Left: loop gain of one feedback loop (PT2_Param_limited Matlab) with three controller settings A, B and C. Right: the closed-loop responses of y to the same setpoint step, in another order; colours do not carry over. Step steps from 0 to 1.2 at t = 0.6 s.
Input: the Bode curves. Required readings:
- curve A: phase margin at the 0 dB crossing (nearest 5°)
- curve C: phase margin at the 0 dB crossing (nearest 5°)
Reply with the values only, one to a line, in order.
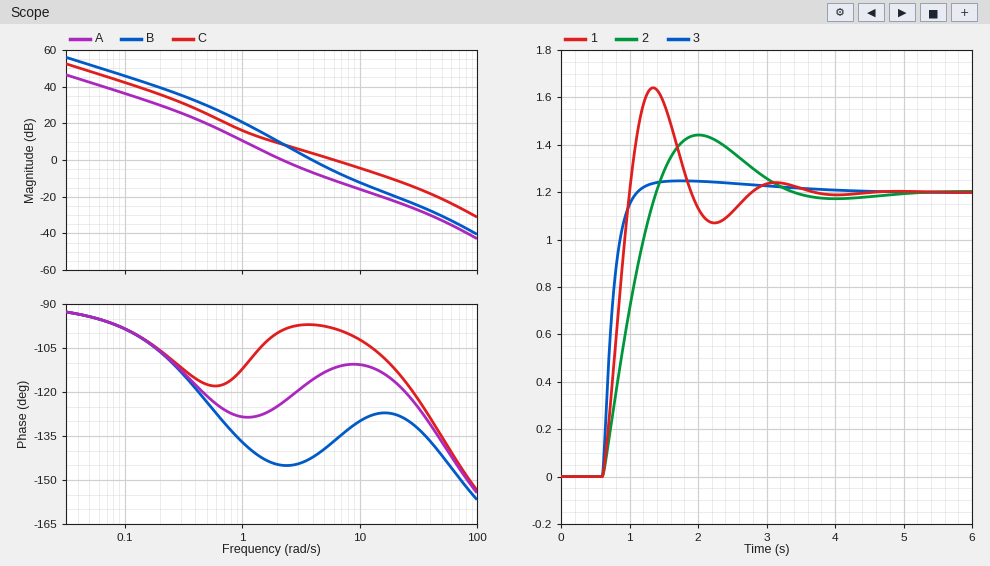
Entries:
55°
80°
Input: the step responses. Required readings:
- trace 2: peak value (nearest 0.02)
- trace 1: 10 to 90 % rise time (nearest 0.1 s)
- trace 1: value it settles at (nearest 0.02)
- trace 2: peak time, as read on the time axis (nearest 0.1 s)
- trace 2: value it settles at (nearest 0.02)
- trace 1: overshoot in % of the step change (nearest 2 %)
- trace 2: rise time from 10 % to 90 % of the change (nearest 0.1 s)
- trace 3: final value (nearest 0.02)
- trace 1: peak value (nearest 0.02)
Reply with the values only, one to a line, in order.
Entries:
1.44
0.3 s
1.20
2.0 s
1.20
36 %
0.6 s
1.20
1.64
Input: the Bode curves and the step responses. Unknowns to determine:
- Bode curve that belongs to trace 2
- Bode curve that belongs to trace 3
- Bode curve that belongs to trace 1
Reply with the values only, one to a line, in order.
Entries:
A
C
B
